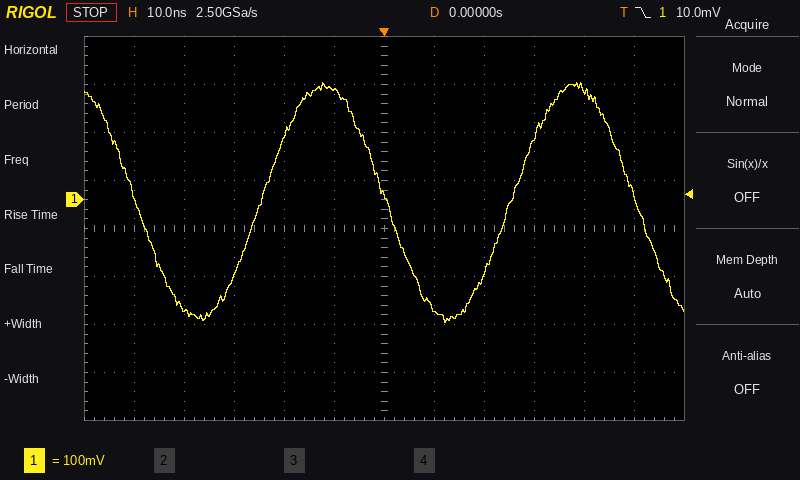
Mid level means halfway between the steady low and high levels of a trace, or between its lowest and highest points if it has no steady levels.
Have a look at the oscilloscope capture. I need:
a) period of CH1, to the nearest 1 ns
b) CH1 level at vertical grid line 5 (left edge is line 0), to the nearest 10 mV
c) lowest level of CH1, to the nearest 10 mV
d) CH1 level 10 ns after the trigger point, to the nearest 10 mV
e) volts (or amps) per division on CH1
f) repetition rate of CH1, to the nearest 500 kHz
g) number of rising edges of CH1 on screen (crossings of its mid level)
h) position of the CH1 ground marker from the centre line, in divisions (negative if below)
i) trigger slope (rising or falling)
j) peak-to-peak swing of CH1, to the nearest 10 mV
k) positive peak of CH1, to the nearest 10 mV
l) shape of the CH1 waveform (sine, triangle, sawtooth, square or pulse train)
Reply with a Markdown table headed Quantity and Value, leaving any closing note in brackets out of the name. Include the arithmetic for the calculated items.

| Quantity | Value |
|---|---|
| period of CH1, to the nearest 1 ns | 50 ns |
| CH1 level at vertical grid line 5 (left edge is line 0), to the nearest 10 mV | 230 mV |
| lowest level of CH1, to the nearest 10 mV | -260 mV |
| CH1 level 10 ns after the trigger point, to the nearest 10 mV | -230 mV |
| volts (or amps) per division on CH1 | 100 mV |
| repetition rate of CH1, to the nearest 500 kHz | 1 / 50 ns ≈ 20.0 MHz |
| number of rising edges of CH1 on screen | 2 |
| position of the CH1 ground marker from the centre line, in divisions | +0.6 div |
| trigger slope | falling |
| peak-to-peak swing of CH1, to the nearest 10 mV | 240 mV − (-260 mV) = 500 mV |
| positive peak of CH1, to the nearest 10 mV | 240 mV |
| shape of the CH1 waveform | sine |
